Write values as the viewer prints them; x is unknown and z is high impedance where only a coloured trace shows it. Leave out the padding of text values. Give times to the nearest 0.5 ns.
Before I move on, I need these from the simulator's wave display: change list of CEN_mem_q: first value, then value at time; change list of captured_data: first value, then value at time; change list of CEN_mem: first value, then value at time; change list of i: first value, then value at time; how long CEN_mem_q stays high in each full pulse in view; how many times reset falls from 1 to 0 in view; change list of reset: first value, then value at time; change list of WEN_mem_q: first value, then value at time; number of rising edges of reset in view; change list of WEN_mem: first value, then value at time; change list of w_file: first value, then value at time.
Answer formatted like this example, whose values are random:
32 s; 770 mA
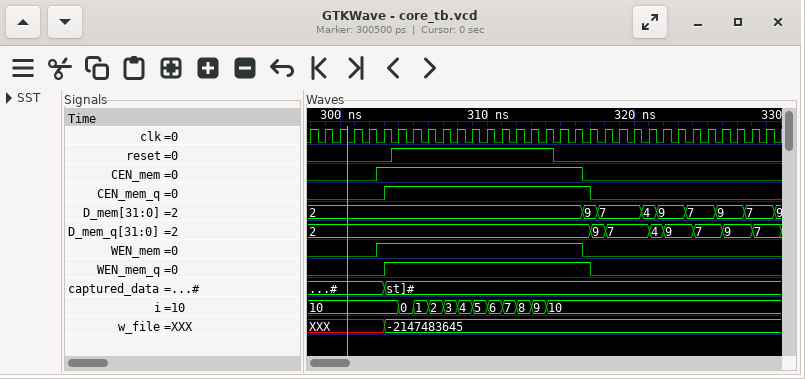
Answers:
0, 1 at 303 ns, 0 at 317 ns; #, st]# at 303 ns; 0, 1 at 302.5 ns, 0 at 316.5 ns; 10, 0 at 304 ns, 1 at 305 ns, 2 at 306 ns, 3 at 307 ns, 4 at 308 ns, 5 at 309 ns, 6 at 310 ns, 7 at 311 ns, 8 at 312 ns, 9 at 313 ns, 10 at 314 ns; 14 ns; 1; 0, 1 at 303.5 ns, 0 at 314.5 ns; 0, 1 at 303 ns, 0 at 317 ns; 1; 0, 1 at 302.5 ns, 0 at 316.5 ns; XXX, -2147483645 at 303 ns
